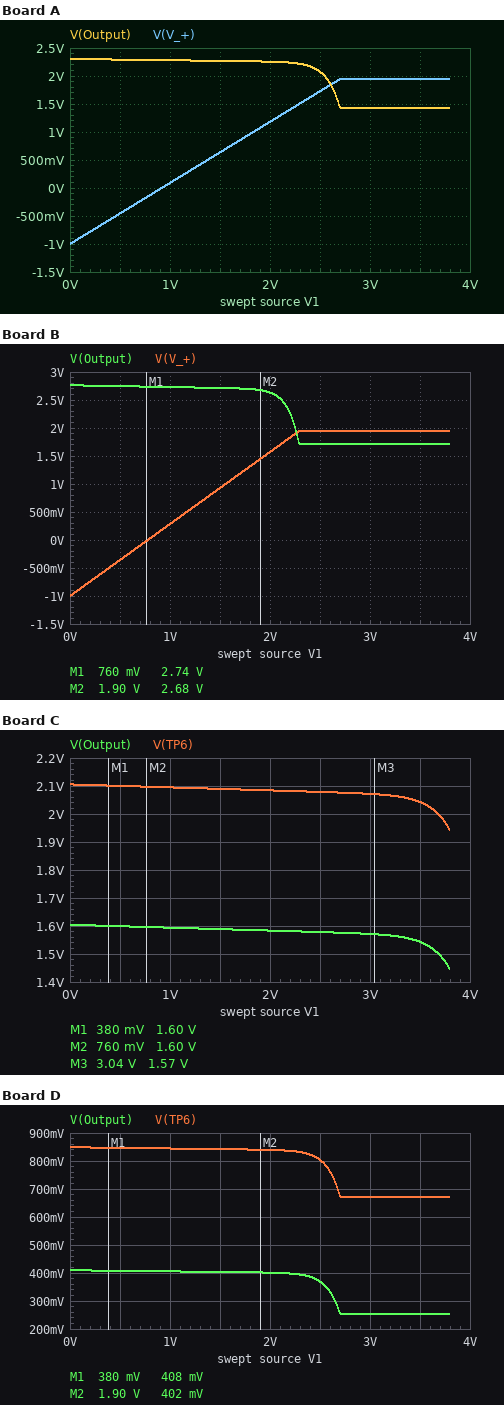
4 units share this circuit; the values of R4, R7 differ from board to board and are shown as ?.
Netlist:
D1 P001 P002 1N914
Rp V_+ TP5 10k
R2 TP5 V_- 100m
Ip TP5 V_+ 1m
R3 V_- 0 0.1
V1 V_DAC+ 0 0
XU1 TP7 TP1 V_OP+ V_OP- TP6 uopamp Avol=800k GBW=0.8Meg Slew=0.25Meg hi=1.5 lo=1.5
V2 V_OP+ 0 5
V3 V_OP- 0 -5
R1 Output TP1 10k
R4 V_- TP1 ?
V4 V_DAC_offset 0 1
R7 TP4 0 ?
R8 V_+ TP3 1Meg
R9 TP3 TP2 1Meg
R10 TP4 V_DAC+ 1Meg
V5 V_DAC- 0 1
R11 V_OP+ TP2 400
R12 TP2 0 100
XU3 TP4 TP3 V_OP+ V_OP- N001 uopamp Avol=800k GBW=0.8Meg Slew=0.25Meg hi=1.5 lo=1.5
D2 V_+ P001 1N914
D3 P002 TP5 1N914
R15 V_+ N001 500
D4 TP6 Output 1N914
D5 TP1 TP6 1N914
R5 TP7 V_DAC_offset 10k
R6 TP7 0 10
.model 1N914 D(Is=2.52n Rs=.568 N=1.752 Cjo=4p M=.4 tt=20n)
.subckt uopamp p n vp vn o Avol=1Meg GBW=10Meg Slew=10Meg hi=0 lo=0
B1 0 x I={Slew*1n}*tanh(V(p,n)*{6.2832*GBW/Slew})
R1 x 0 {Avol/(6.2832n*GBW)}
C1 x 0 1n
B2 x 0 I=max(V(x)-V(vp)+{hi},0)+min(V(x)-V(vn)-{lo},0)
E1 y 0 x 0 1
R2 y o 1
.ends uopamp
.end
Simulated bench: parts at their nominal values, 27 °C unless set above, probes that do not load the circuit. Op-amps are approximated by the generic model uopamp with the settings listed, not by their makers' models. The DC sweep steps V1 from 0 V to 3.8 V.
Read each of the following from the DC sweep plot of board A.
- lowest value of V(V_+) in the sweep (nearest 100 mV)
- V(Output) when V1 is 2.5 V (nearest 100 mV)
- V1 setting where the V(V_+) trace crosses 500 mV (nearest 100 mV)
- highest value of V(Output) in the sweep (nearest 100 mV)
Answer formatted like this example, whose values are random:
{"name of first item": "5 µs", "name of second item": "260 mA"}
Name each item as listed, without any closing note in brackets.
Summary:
{"lowest value of V(V_+) in the sweep": "-1.0 V", "V(Output) when V1 is 2.5 V": "2.1 V", "V1 setting where the V(V_+) trace crosses 500 mV": "1.4 V", "highest value of V(Output) in the sweep": "2.3 V"}
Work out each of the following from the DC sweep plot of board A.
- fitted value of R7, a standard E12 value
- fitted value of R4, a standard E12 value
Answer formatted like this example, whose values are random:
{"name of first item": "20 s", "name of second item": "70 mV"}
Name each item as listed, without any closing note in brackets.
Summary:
{"fitted value of R7, a standard E12 value": "1.2 MΩ", "fitted value of R4, a standard E12 value": "4.7 Ω"}
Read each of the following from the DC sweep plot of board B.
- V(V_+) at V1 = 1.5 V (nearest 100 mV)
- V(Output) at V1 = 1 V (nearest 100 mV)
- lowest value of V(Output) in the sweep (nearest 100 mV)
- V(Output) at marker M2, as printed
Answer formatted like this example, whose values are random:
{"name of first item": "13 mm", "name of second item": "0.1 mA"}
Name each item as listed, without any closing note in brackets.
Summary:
{"V(V_+) at V1 = 1.5 V": "900 mV", "V(Output) at V1 = 1 V": "2.7 V", "lowest value of V(Output) in the sweep": "1.7 V", "V(Output) at marker M2, as printed": "2.68 V"}
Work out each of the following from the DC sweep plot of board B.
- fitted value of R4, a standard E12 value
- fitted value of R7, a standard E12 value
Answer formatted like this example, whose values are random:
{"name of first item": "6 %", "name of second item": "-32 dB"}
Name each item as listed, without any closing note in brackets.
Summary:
{"fitted value of R4, a standard E12 value": "3.9 Ω", "fitted value of R7, a standard E12 value": "1.8 MΩ"}
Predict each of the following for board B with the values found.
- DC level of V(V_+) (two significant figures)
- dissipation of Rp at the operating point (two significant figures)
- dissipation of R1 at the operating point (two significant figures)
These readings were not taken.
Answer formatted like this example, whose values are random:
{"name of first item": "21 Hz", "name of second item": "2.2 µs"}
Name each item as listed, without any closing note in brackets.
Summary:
{"DC level of V(V_+)": "-1.0 V", "dissipation of Rp at the operating point": "100 µW", "dissipation of R1 at the operating point": "760 µW"}
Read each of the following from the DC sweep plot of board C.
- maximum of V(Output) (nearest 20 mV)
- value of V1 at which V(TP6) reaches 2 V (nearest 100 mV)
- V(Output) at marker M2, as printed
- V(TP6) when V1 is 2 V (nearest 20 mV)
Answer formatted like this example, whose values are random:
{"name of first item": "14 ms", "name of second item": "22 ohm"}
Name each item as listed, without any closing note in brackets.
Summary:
{"maximum of V(Output)": "1.60 V", "value of V1 at which V(TP6) reaches 2 V": "3.7 V", "V(Output) at marker M2, as printed": "1.60 V", "V(TP6) when V1 is 2 V": "2.08 V"}
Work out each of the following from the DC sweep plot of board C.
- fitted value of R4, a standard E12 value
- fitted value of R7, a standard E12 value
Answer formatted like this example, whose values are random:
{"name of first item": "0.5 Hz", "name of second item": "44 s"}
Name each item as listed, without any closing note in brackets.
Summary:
{"fitted value of R4, a standard E12 value": "6.8 Ω", "fitted value of R7, a standard E12 value": "560 kΩ"}
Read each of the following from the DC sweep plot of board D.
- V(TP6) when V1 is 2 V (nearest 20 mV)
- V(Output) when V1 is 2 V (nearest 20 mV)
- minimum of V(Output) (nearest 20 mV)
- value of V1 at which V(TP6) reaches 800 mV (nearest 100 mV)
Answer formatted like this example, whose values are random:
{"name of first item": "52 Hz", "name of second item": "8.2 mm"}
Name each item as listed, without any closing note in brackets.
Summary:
{"V(TP6) when V1 is 2 V": "840 mV", "V(Output) when V1 is 2 V": "400 mV", "minimum of V(Output)": "260 mV", "value of V1 at which V(TP6) reaches 800 mV": "2.5 V"}
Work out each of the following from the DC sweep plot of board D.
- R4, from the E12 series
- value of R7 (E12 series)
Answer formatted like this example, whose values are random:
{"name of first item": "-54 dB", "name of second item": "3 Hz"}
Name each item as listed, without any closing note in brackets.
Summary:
{"R4, from the E12 series": "27 Ω", "value of R7": "1.2 MΩ"}
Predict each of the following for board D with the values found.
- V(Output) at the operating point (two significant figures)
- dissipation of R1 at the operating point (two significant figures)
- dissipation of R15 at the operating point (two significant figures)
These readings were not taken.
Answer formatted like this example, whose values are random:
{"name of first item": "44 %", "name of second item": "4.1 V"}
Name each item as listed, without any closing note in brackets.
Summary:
{"V(Output) at the operating point": "410 mV", "dissipation of R1 at the operating point": "17 µW", "dissipation of R15 at the operating point": "610 µW"}
